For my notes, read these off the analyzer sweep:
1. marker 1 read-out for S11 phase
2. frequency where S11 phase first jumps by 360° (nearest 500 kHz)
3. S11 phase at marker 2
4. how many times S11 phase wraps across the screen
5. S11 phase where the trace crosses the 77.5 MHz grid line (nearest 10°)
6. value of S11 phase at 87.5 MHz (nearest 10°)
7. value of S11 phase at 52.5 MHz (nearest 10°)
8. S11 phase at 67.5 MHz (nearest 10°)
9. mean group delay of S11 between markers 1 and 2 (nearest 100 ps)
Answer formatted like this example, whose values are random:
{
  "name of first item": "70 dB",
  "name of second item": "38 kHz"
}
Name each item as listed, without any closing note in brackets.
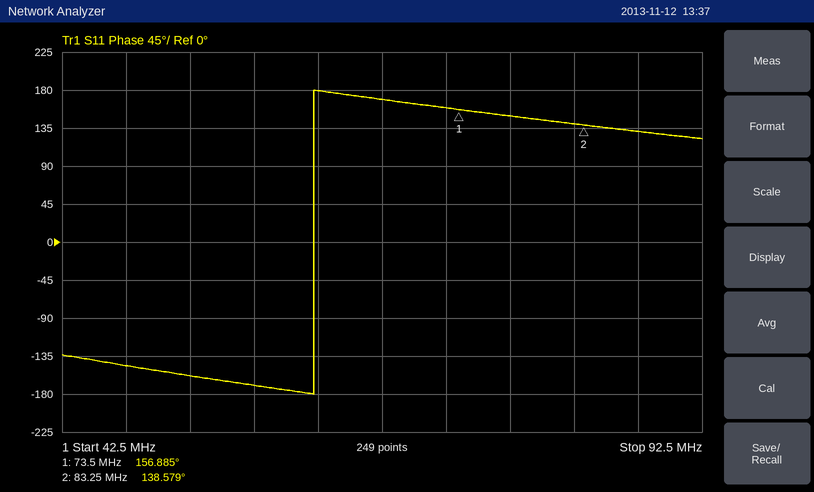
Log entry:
{
  "marker 1 read-out for S11 phase": "156.885°",
  "frequency where S11 phase first jumps by 360°": "62.0 MHz",
  "S11 phase at marker 2": "138.579°",
  "how many times S11 phase wraps across the screen": "1",
  "S11 phase where the trace crosses the 77.5 MHz grid line": "150°",
  "value of S11 phase at 87.5 MHz": "130°",
  "value of S11 phase at 52.5 MHz": "-160°",
  "S11 phase at 67.5 MHz": "170°",
  "mean group delay of S11 between markers 1 and 2": "5.2 ns"
}
